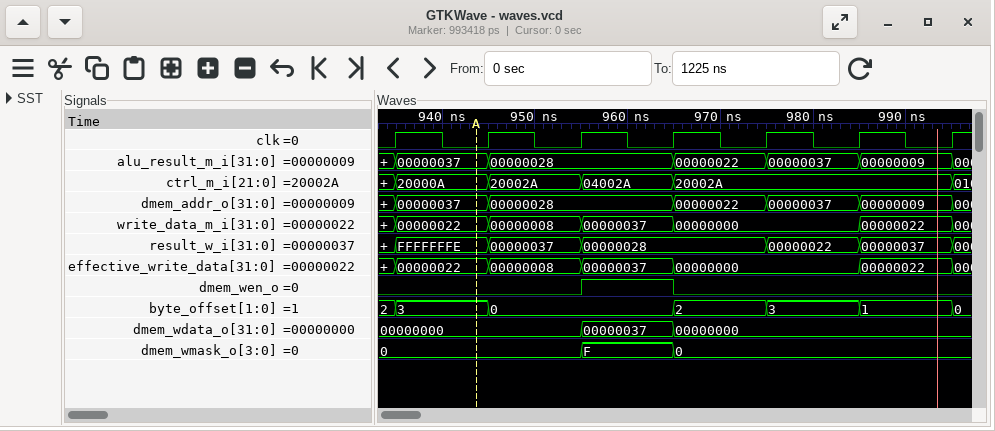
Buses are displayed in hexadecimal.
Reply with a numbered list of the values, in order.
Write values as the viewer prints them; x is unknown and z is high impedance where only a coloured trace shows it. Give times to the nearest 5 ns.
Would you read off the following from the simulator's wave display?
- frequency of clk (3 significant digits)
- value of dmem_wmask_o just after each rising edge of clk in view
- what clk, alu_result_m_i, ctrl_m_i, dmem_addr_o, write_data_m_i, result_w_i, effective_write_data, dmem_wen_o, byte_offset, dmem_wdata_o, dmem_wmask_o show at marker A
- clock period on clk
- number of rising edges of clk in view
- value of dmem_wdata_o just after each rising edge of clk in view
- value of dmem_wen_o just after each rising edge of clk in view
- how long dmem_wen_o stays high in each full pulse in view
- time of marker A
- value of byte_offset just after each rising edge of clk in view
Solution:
1. 100 MHz
2. 0, 0, F, 0, 0, 0, 0
3. clk=0, alu_result_m_i=00000037, ctrl_m_i=20000A, dmem_addr_o=00000037, write_data_m_i=00000022, result_w_i=FFFFFFFE, effective_write_data=00000022, dmem_wen_o=0, byte_offset=3, dmem_wdata_o=00000000, dmem_wmask_o=0
4. 10 ns
5. 7
6. 00000000, 00000000, 00000037, 00000000, 00000000, 00000000, 00000000
7. 0 0 1 0 0 0 0
8. 10 ns
9. 945 ns
10. 3, 0, 0, 2, 3, 1, 0
